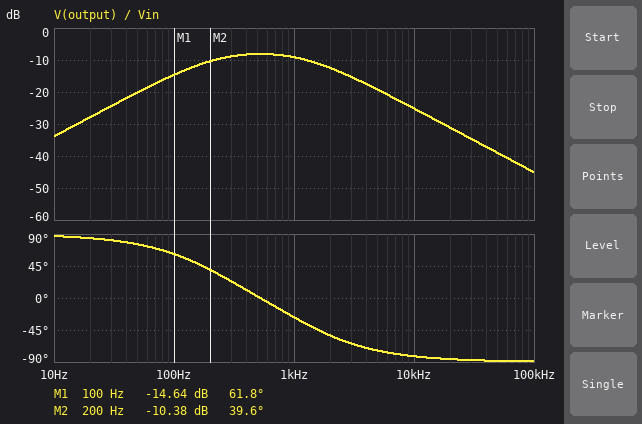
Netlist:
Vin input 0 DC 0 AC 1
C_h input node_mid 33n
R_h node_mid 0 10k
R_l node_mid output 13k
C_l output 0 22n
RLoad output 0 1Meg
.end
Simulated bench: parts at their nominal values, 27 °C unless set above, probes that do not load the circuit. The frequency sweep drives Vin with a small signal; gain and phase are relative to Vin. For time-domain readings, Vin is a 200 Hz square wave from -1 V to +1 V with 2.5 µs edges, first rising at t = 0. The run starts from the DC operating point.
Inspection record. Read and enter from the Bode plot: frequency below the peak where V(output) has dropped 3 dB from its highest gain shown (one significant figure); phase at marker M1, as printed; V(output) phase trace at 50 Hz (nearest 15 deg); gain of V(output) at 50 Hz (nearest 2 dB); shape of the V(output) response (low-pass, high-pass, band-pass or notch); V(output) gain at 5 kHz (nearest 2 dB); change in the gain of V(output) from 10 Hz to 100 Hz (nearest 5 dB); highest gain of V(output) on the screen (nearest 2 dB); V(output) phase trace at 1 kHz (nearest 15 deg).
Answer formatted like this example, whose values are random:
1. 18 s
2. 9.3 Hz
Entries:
1. 200 Hz
2. 61.8 deg
3. 75 deg
4. -20 dB
5. band-pass
6. -20 dB
7. 20 dB
8. -8 dB
9. -30 deg
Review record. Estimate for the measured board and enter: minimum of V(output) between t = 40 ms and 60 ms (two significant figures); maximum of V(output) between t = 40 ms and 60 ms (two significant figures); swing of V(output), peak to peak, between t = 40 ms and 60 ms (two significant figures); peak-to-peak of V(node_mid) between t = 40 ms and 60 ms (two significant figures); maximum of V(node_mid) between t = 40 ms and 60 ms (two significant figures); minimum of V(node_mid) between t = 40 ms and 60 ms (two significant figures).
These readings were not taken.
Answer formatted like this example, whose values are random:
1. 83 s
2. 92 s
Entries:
1. -610 mV
2. 610 mV
3. 1.2 V
4. 3.9 V
5. 2.0 V
6. -2.0 V
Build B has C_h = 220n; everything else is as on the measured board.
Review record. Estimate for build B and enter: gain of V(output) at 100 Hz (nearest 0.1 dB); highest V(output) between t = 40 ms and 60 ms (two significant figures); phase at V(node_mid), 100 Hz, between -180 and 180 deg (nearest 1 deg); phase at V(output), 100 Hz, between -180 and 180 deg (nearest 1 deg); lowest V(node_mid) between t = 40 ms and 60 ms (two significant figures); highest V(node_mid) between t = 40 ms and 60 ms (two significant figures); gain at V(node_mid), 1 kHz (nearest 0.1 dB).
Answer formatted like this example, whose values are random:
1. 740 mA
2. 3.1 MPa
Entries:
1. -2.7 dB
2. 970 mV
3. 34 deg
4. 24 deg
5. -1.5 V
6. 1.5 V
7. -0.3 dB
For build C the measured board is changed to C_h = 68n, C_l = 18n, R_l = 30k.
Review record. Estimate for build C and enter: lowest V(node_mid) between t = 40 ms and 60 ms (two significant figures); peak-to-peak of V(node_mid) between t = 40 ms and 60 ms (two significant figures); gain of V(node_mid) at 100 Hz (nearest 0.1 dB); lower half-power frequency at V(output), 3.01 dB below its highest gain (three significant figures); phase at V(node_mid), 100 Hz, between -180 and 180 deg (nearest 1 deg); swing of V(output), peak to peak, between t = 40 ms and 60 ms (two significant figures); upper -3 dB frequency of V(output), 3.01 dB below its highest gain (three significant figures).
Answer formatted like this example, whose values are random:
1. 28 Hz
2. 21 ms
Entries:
1. -1.9 V
2. 3.8 V
3. -8.7 dB
4. 100 Hz
5. 63 deg
6. 1.3 V
7. 716 Hz
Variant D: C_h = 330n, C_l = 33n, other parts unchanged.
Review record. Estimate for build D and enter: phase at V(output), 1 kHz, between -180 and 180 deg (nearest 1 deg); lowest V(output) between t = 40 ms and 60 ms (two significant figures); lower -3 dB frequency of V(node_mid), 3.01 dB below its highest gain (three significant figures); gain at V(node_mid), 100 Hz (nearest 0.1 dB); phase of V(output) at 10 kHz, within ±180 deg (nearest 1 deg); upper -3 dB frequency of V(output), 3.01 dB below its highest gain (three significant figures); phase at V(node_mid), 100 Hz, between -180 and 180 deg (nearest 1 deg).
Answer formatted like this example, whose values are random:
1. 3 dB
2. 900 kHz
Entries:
1. -65 deg
2. -870 mV
3. 55.3 Hz
4. -1.6 dB
5. -87 deg
6. 498 Hz
7. 25 deg
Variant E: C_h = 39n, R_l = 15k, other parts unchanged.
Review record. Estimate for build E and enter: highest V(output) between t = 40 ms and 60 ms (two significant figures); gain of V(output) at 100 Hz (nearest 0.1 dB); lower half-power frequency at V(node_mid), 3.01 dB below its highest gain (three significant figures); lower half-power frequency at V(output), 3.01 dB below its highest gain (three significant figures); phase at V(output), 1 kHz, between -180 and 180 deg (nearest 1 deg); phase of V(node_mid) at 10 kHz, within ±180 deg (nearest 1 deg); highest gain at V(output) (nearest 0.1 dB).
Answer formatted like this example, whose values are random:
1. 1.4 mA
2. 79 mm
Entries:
1. 630 mV
2. -13.4 dB
3. 747 Hz
4. 153 Hz
5. -34 deg
6. 4 deg
7. -7.7 dB
